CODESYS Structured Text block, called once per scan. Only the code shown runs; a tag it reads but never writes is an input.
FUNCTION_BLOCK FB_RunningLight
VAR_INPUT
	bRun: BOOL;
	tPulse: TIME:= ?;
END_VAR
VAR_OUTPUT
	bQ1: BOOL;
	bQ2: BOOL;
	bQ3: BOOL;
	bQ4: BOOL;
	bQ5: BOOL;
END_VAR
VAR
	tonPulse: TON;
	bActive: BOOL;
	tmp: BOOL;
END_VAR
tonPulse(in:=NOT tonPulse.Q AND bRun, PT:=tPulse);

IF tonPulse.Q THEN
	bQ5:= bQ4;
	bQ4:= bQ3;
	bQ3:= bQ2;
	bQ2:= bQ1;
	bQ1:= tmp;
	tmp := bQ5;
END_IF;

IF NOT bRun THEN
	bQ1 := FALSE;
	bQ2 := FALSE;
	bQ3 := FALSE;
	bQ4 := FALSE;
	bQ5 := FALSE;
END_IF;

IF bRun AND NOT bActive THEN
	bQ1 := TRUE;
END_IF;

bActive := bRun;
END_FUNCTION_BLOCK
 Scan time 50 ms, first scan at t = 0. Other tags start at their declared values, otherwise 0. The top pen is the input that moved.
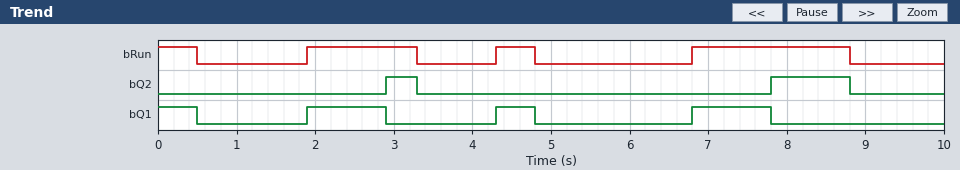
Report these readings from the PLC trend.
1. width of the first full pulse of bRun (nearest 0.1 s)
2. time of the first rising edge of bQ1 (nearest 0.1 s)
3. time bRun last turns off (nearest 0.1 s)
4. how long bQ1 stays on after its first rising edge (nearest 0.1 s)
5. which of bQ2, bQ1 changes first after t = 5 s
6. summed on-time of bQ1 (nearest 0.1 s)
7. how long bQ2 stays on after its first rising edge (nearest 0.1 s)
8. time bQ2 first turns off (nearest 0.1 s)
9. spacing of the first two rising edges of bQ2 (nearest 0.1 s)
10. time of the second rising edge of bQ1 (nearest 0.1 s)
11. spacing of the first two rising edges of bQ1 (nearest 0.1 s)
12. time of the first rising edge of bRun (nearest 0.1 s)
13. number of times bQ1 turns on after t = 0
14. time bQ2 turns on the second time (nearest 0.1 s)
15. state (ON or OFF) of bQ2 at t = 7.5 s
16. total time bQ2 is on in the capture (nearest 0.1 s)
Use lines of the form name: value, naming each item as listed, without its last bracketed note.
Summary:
width of the first full pulse of bRun: 1.4 s
time of the first rising edge of bQ1: 1.9 s
time bRun last turns off: 8.8 s
how long bQ1 stays on after its first rising edge: 1.0 s
which of bQ2, bQ1 changes first after t = 5 s: bQ1
summed on-time of bQ1: 3.0 s
how long bQ2 stays on after its first rising edge: 0.4 s
time bQ2 first turns off: 3.3 s
spacing of the first two rising edges of bQ2: 4.9 s
time of the second rising edge of bQ1: 4.3 s
spacing of the first two rising edges of bQ1: 2.4 s
time of the first rising edge of bRun: 1.9 s
number of times bQ1 turns on after t = 0: 3
time bQ2 turns on the second time: 7.8 s
state (ON or OFF) of bQ2 at t = 7.5 s: OFF
total time bQ2 is on in the capture: 1.4 s
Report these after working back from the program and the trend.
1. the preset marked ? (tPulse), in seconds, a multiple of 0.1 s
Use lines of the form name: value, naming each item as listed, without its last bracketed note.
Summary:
the preset marked ? (tPulse), in seconds, a multiple of 0.1 s: 1.0 s
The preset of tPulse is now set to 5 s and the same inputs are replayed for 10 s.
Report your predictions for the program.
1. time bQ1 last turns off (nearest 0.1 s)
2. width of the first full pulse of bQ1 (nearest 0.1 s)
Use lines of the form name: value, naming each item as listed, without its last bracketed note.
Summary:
time bQ1 last turns off: 8.8 s
width of the first full pulse of bQ1: 1.4 s
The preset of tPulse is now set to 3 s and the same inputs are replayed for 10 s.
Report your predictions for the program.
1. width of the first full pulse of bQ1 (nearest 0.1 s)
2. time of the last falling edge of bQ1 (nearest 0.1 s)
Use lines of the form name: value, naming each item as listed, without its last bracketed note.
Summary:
width of the first full pulse of bQ1: 1.4 s
time of the last falling edge of bQ1: 8.8 s
